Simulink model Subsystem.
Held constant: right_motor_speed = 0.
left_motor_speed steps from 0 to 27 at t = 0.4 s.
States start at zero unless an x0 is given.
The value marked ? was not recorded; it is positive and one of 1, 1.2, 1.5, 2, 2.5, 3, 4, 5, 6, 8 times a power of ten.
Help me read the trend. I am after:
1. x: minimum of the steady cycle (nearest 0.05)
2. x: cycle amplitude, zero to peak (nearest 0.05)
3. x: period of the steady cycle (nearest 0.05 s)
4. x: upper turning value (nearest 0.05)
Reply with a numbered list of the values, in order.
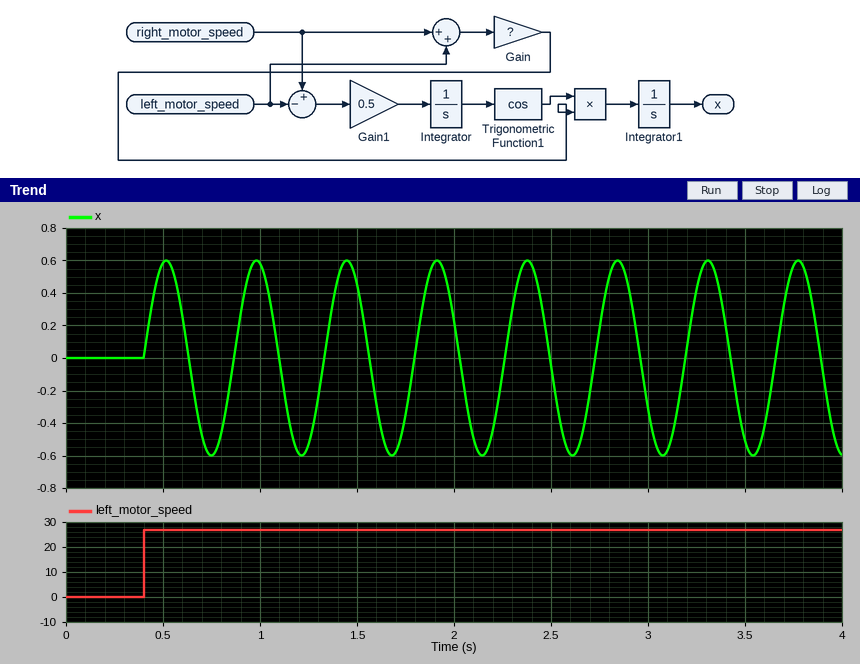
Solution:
1. -0.60
2. 0.60
3. 0.45 s
4. 0.60
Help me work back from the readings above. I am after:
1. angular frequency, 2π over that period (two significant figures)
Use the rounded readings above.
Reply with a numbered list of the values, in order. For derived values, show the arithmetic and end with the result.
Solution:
1. 2π / 0.45 = 14 rad/s
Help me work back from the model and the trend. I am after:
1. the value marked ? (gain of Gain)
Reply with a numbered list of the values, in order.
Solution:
1. 0.3
